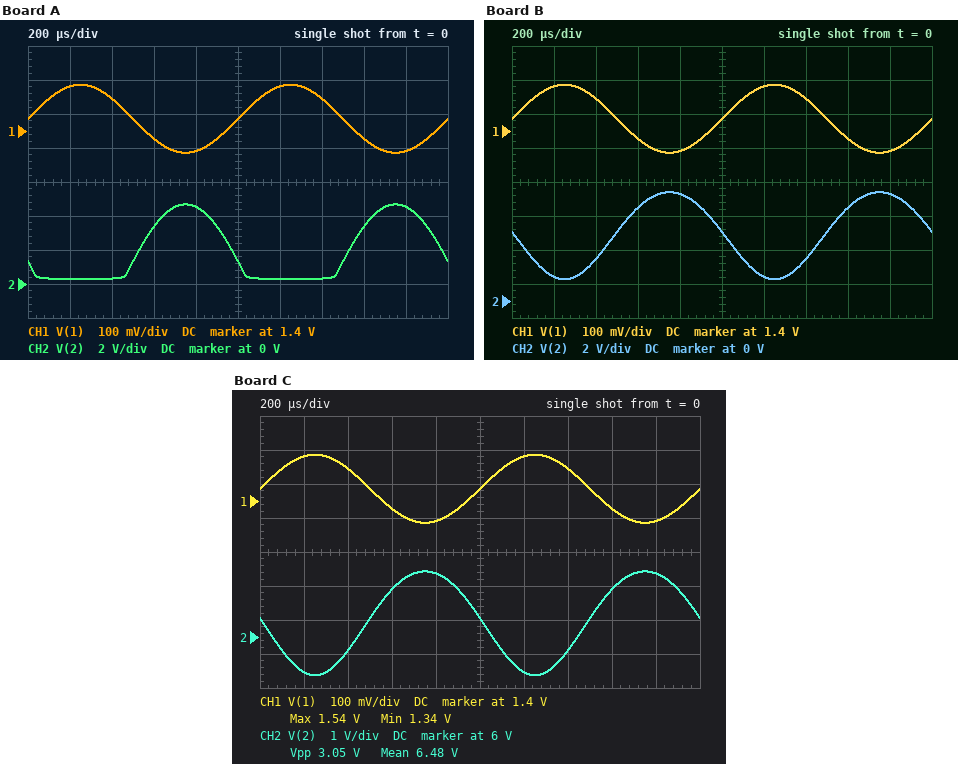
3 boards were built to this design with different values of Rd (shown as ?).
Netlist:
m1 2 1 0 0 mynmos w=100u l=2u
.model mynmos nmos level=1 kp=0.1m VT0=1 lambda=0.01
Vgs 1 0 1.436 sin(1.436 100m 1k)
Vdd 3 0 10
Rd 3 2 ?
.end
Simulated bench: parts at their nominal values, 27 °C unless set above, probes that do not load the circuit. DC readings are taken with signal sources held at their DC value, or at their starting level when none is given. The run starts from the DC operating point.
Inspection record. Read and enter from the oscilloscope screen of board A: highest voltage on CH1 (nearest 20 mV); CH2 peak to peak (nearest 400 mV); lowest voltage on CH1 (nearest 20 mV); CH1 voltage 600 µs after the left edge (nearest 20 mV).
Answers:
1.54 V
4.4 V
1.34 V
1.38 V
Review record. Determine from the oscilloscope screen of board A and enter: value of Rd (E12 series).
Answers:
18 kΩ
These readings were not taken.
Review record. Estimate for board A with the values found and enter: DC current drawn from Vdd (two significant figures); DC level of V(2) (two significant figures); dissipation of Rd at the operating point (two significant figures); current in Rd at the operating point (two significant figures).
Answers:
480 µA
1.3 V
4.2 mW
480 µA
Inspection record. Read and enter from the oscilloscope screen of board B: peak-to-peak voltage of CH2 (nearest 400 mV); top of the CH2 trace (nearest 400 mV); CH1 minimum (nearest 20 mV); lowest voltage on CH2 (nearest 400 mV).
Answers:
5.2 V
6.4 V
1.34 V
1.2 V
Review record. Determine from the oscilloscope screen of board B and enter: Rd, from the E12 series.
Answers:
12 kΩ
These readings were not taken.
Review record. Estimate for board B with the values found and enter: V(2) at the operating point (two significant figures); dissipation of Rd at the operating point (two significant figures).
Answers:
4.1 V
2.9 mW
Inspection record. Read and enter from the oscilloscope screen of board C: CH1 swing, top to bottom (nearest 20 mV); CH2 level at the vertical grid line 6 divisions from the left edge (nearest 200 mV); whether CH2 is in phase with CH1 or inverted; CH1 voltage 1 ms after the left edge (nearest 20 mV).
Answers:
200 mV
5.0 V
inverted
1.44 V
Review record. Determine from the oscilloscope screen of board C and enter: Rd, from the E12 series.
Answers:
6.8 kΩ
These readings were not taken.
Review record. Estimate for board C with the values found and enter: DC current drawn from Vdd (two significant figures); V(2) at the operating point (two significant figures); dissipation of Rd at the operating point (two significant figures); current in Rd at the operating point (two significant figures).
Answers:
510 µA
6.6 V
1.7 mW
510 µA
